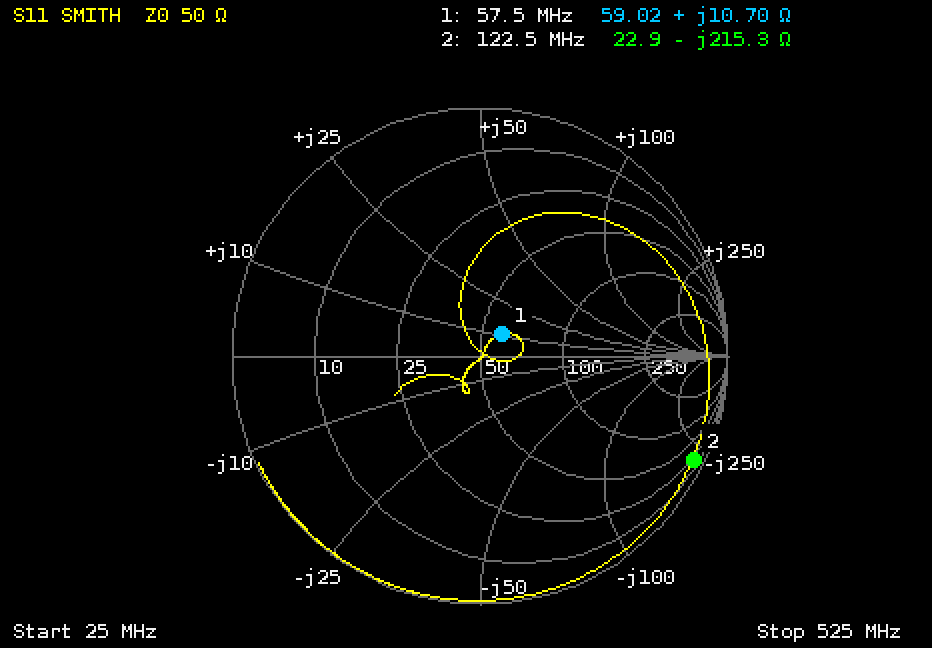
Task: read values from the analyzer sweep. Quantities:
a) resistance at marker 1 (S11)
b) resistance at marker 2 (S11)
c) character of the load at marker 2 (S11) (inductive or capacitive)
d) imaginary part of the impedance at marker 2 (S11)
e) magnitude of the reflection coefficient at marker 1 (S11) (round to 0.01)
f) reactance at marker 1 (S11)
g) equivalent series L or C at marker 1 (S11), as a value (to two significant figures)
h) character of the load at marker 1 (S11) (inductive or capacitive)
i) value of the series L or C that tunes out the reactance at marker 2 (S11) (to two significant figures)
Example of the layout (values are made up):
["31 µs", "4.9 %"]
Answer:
["59.02 Ω", "22.9 Ω", "capacitive", "-215.3 Ω", "0.13", "+10.70 Ω", "30 nH", "inductive", "280 nH"]
